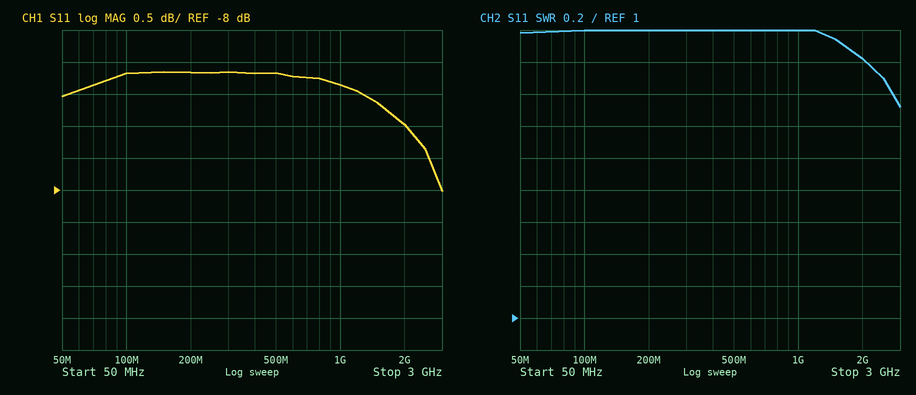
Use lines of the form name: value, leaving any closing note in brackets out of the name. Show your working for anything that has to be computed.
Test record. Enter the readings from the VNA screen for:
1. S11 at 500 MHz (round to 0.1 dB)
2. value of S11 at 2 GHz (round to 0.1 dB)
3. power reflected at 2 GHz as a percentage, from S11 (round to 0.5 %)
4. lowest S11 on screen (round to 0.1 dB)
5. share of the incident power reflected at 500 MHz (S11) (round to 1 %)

S11 at 500 MHz: -6.2 dB
value of S11 at 2 GHz: -7.0 dB
power reflected at 2 GHz as a percentage, from S11: 10^(-7/10) ≈ 20.0 %
lowest S11 on screen: -8.0 dB
share of the incident power reflected at 500 MHz (S11): 10^(-6.2/10) ≈ 24 %
